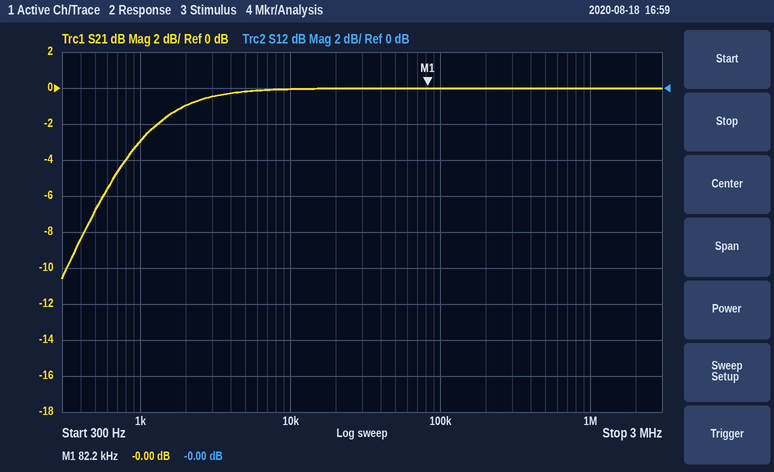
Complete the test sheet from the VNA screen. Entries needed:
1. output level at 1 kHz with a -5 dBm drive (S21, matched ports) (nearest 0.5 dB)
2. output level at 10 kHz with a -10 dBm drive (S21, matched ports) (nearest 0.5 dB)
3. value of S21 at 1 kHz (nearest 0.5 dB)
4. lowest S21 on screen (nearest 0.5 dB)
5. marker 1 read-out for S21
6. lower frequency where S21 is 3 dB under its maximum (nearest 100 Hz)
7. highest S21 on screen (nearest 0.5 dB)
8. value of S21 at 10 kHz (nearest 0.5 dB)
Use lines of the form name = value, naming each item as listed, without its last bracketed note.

output level at 1 kHz with a -5 dBm drive (S21, matched ports) = -8.0 dBm
output level at 10 kHz with a -10 dBm drive (S21, matched ports) = -10.0 dBm
value of S21 at 1 kHz = -3.0 dB
lowest S21 on screen = -10.5 dB
marker 1 read-out for S21 = -0.00 dB
lower frequency where S21 is 3 dB under its maximum = 1.0 kHz
highest S21 on screen = 0.0 dB
value of S21 at 10 kHz = 0.0 dB
